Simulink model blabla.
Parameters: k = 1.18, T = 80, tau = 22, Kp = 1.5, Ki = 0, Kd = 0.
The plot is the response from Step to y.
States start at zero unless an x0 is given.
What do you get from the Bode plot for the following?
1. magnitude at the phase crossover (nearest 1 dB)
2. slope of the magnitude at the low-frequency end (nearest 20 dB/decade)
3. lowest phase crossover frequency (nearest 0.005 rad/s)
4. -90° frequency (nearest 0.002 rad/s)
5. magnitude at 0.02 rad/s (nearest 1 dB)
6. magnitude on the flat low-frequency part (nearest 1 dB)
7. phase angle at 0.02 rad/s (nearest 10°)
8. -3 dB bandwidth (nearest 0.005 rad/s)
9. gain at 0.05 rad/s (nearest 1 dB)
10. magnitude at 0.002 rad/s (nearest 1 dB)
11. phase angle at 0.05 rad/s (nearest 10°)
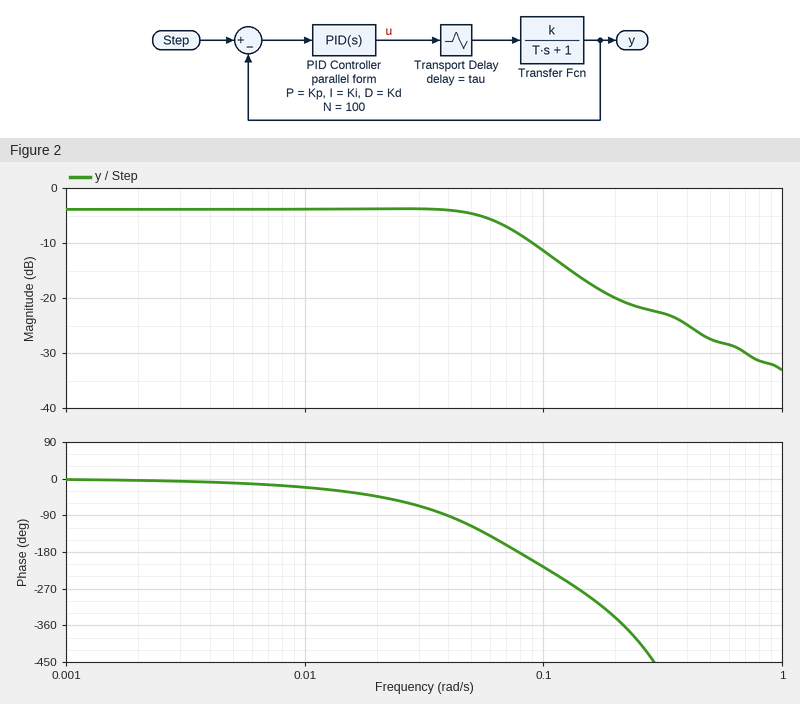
-8 dB
0 dB/decade
0.080 rad/s
0.040 rad/s
-4 dB
-4 dB
-40°
0.070 rad/s
-5 dB
-4 dB
-120°
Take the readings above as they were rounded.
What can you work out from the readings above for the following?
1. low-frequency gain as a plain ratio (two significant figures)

0.63
